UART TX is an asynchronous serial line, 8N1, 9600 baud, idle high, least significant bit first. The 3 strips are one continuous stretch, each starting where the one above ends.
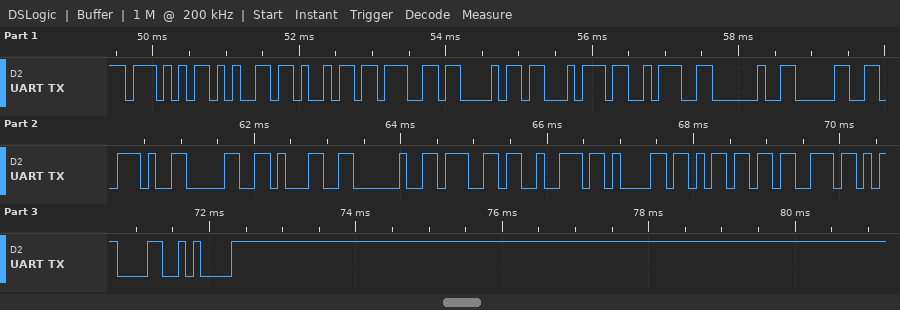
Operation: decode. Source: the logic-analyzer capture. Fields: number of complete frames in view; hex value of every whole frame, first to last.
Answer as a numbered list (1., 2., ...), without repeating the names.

1. 20
2. 0x57 0x65 0x69 0x67 0x68 0x74 0x3A 0x20 0x30 0x2E 0x30 0x31 0x20 0x67 0x72 0x61 0x6D 0x73 0x0D 0x0A
